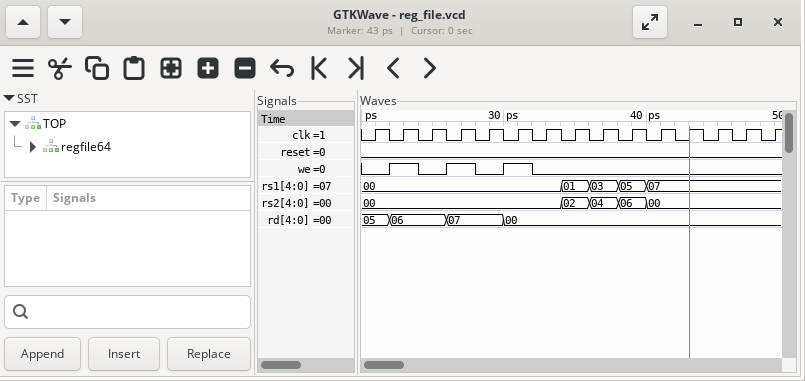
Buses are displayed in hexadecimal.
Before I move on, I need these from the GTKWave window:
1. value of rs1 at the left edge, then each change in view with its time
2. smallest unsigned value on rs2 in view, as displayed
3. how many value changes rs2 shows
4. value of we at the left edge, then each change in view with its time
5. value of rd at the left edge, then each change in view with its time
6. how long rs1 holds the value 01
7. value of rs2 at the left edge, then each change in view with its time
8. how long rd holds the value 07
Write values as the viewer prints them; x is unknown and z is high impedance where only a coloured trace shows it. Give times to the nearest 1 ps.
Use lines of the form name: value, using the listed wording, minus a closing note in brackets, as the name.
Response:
value of rs1 at the left edge, then each change in view with its time: 00, 01 at 34 ps, 03 at 36 ps, 05 at 38 ps, 07 at 40 ps
smallest unsigned value on rs2 in view, as displayed: 00
how many value changes rs2 shows: 4
value of we at the left edge, then each change in view with its time: 0, 1 at 22 ps, 0 at 24 ps, 1 at 26 ps, 0 at 28 ps, 1 at 30 ps, 0 at 32 ps
value of rd at the left edge, then each change in view with its time: 05, 06 at 22 ps, 07 at 26 ps, 00 at 30 ps
how long rs1 holds the value 01: 2 ps
value of rs2 at the left edge, then each change in view with its time: 00, 02 at 34 ps, 04 at 36 ps, 06 at 38 ps, 00 at 40 ps
how long rd holds the value 07: 4 ps
